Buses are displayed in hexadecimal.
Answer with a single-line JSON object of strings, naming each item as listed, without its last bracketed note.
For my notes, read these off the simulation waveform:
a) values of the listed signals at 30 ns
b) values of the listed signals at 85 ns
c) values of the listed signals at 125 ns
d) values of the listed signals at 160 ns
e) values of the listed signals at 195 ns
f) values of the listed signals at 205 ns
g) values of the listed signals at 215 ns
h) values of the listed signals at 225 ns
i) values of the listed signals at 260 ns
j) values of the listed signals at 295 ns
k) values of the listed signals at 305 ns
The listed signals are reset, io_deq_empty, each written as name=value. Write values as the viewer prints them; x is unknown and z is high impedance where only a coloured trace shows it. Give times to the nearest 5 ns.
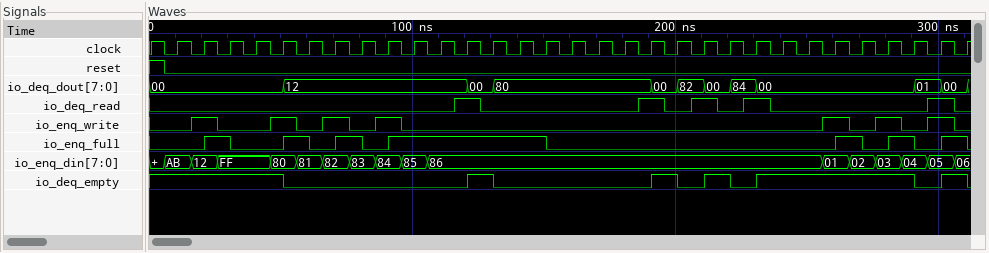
{"values of the listed signals at 30 ns": "reset=0, io_deq_empty=1", "values of the listed signals at 85 ns": "reset=0, io_deq_empty=0", "values of the listed signals at 125 ns": "reset=0, io_deq_empty=1", "values of the listed signals at 160 ns": "reset=0, io_deq_empty=0", "values of the listed signals at 195 ns": "reset=0, io_deq_empty=1", "values of the listed signals at 205 ns": "reset=0, io_deq_empty=0", "values of the listed signals at 215 ns": "reset=0, io_deq_empty=1", "values of the listed signals at 225 ns": "reset=0, io_deq_empty=0", "values of the listed signals at 260 ns": "reset=0, io_deq_empty=1", "values of the listed signals at 295 ns": "reset=0, io_deq_empty=0", "values of the listed signals at 305 ns": "reset=0, io_deq_empty=1"}
